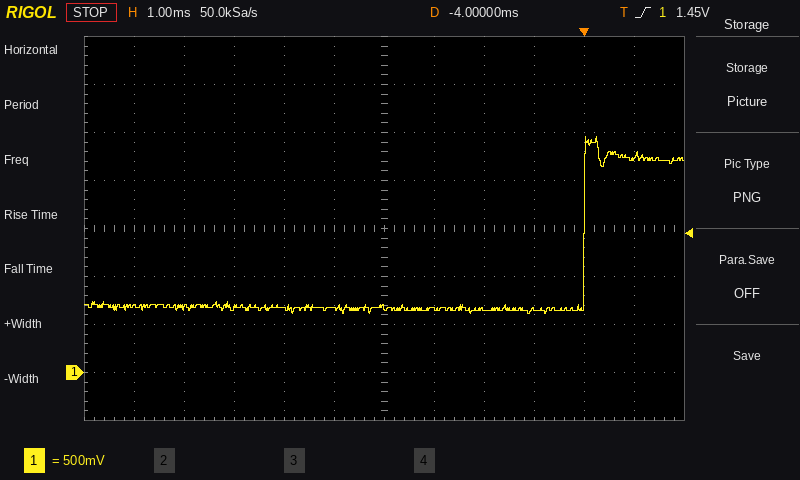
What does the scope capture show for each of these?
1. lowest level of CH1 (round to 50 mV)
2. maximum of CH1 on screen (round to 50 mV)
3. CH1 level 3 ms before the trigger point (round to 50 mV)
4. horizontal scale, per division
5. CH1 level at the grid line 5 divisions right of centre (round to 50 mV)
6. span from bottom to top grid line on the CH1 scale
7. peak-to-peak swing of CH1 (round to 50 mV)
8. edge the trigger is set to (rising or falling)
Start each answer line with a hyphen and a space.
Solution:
- 600 mV
- 2.45 V
- 650 mV
- 1 ms
- 2.25 V
- 4 V
- 1.85 V
- rising
